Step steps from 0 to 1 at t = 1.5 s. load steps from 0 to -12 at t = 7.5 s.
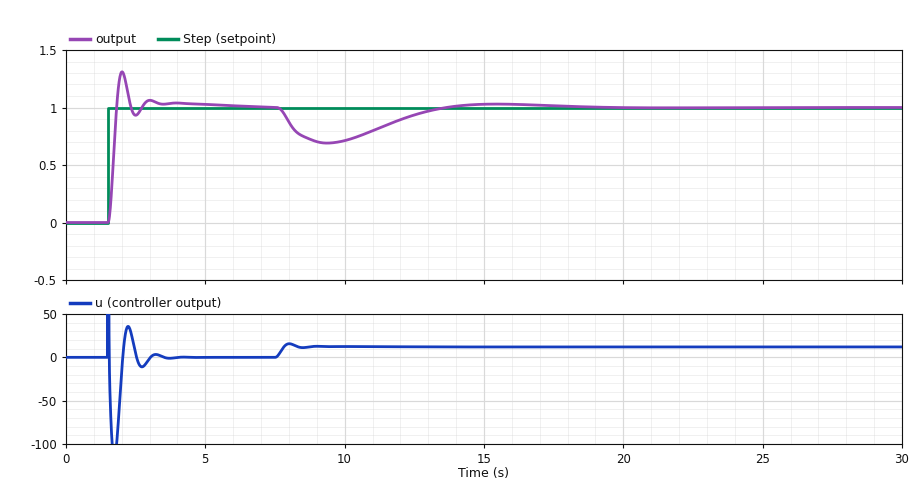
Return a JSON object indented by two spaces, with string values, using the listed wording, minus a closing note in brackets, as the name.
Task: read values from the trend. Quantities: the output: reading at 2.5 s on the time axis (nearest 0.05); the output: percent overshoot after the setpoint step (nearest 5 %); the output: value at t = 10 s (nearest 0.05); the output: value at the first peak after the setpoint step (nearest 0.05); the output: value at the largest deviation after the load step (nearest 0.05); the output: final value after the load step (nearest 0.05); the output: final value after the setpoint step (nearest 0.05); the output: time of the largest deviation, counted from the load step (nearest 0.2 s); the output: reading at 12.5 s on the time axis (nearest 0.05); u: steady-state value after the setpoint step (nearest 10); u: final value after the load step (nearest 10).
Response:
{
  "the output: reading at 2.5 s on the time axis": "0.95",
  "the output: percent overshoot after the setpoint step": "30 %",
  "the output: value at t = 10 s": "0.70",
  "the output: value at the first peak after the setpoint step": "1.30",
  "the output: value at the largest deviation after the load step": "0.70",
  "the output: final value after the load step": "1.00",
  "the output: final value after the setpoint step": "1.00",
  "the output: time of the largest deviation, counted from the load step": "1.8 s",
  "the output: reading at 12.5 s on the time axis": "0.95",
  "u: steady-state value after the setpoint step": "0",
  "u: final value after the load step": "10"
}
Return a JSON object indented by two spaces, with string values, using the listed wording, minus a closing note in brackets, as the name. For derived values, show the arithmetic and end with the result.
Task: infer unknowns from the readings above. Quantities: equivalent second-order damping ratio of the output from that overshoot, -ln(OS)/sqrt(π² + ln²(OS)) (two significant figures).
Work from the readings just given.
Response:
{
  "equivalent second-order damping ratio of the output from that overshoot, -ln(OS)/sqrt(π² + ln²(OS))": "ln(0.3) = -1.204; 1.204 / sqrt(9.870 + 1.450) = 0.36"
}
